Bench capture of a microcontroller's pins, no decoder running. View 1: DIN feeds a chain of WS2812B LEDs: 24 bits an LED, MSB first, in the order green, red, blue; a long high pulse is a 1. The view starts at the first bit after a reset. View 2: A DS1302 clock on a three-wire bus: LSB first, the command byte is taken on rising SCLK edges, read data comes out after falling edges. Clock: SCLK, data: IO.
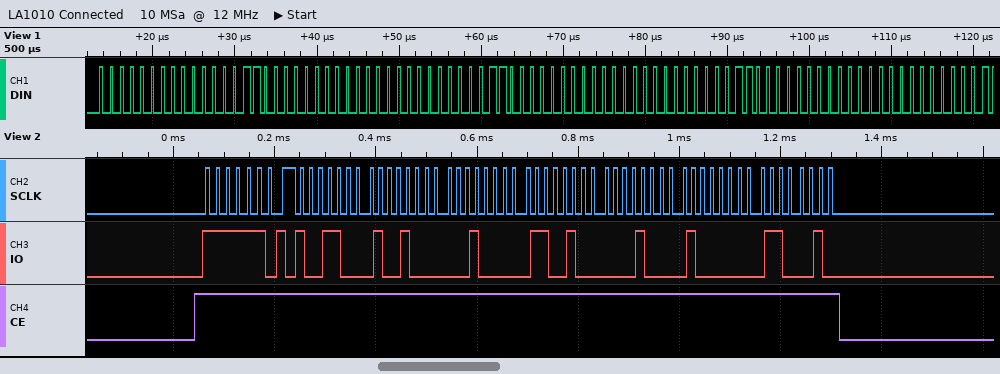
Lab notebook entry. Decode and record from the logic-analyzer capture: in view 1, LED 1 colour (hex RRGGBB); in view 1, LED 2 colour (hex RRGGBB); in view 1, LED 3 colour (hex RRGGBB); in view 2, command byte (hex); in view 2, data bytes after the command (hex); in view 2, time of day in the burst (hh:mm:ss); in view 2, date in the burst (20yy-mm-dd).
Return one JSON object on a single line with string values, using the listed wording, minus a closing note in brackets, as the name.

{"in view 1, LED 1 colour": "#030000", "in view 1, LED 2 colour": "#030000", "in view 1, LED 3 colour": "#030000", "in view 2, command byte": "0xBF", "in view 2, data bytes after the command": "19 09 04 13 08 01 23", "in view 2, time of day in the burst": "04:09:19", "in view 2, date in the burst": "2023-08-13"}
